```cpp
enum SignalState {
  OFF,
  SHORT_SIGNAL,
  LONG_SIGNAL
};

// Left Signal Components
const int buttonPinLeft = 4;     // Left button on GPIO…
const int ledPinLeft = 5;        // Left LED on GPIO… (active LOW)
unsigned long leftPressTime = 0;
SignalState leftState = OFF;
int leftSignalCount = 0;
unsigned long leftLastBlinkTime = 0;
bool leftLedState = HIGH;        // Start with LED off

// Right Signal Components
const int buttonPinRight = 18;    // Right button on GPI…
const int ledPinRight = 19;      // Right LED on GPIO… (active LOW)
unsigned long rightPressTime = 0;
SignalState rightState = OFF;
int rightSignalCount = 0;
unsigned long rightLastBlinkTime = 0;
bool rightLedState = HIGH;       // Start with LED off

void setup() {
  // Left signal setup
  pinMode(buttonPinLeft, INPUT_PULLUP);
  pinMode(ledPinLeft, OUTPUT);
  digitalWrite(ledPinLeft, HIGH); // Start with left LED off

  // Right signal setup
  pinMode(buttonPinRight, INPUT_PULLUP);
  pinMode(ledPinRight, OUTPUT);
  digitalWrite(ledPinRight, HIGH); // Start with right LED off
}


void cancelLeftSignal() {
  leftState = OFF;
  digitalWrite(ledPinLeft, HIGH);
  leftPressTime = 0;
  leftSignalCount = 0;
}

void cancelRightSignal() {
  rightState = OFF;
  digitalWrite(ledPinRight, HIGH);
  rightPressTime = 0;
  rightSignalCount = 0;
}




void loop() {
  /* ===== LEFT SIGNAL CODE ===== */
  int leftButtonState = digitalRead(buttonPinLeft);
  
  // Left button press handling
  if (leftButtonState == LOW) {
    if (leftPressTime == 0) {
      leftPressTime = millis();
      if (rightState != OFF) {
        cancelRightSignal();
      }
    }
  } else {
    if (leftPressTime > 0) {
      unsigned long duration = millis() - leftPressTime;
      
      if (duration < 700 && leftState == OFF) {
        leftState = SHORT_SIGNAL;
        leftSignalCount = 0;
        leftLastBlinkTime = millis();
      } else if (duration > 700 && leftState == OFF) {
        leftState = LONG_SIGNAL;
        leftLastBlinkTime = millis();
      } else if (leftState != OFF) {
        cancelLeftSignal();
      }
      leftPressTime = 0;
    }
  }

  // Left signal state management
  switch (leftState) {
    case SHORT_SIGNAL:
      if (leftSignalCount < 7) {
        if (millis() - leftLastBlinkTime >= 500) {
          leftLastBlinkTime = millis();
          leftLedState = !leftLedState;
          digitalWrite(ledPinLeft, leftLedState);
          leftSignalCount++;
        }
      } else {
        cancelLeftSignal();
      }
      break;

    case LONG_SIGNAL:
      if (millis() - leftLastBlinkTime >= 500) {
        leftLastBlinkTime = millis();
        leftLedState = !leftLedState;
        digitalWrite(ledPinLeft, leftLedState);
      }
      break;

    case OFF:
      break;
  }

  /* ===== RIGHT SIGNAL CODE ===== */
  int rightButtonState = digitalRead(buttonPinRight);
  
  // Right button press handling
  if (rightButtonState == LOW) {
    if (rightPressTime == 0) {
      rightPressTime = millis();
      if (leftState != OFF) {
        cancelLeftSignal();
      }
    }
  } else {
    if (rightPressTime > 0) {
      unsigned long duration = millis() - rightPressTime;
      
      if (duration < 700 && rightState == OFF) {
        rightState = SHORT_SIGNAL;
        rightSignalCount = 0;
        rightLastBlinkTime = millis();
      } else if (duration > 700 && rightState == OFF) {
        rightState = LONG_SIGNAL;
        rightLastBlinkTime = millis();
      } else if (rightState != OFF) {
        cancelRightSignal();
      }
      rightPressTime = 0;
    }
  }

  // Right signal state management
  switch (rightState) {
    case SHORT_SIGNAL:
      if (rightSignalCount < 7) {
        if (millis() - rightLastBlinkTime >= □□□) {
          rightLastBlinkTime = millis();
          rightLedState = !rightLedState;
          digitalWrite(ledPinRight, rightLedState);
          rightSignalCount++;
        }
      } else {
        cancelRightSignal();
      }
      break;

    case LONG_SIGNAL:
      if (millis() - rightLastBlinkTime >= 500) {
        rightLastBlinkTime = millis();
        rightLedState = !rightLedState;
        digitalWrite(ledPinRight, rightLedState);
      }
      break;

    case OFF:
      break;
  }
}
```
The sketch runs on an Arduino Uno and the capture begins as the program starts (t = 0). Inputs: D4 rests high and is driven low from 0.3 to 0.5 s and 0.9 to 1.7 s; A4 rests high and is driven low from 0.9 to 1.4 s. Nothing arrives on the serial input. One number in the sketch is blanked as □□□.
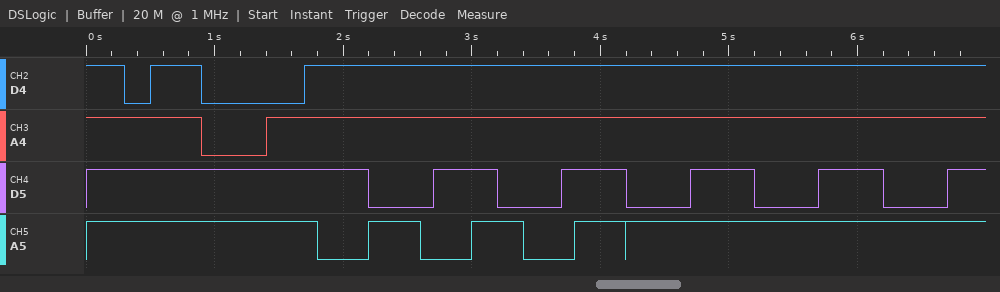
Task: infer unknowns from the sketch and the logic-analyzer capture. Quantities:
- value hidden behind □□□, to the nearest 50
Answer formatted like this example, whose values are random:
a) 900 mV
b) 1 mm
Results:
a) 400
